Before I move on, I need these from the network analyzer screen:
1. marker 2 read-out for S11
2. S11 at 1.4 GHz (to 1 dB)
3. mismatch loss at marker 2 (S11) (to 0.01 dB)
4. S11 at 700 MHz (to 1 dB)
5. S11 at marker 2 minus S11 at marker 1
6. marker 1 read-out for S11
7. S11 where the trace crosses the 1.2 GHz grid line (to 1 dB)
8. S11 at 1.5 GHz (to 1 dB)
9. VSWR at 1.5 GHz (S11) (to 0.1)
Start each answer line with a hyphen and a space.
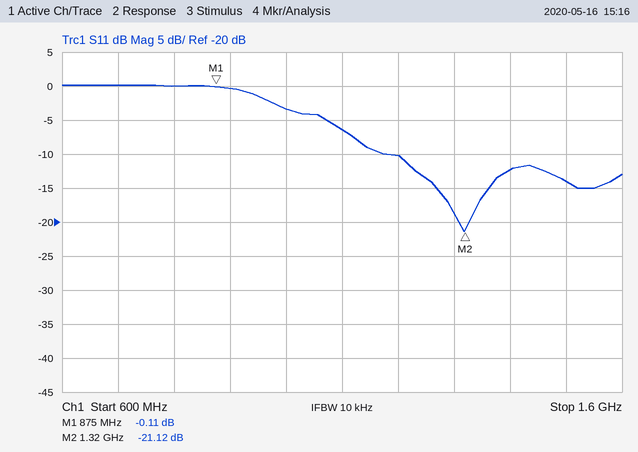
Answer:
- -21.12 dB
- -12 dB
- 0.03 dB
- 0 dB
- -21.01 dB
- -0.11 dB
- -10 dB
- -14 dB
- 1.5
